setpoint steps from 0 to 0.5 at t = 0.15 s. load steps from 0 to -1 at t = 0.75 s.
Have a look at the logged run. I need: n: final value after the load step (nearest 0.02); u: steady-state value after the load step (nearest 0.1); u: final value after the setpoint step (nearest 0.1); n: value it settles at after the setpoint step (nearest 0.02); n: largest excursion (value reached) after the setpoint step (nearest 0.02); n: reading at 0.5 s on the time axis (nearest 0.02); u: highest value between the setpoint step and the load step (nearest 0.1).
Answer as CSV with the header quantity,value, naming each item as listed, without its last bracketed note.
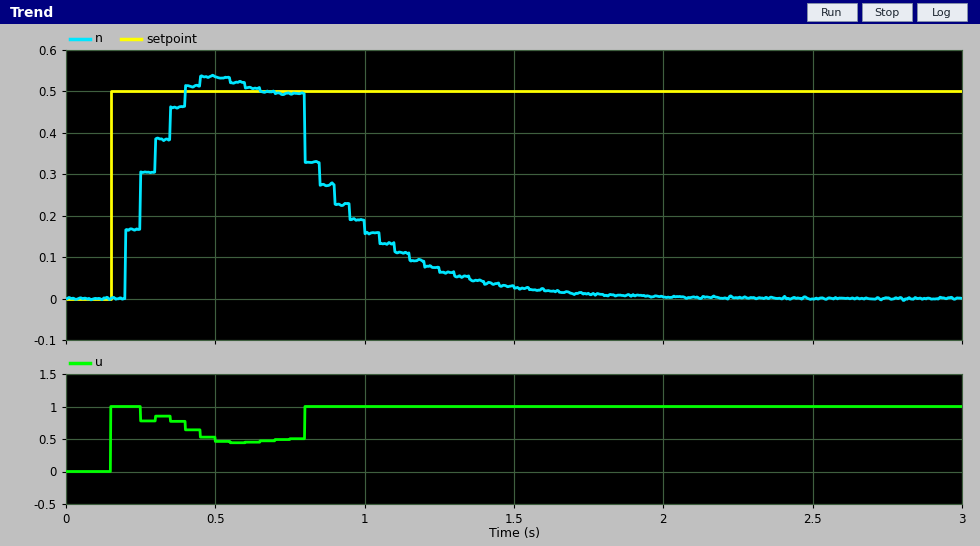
quantity,value
n: final value after the load step,0.00
u: steady-state value after the load step,1.0
u: final value after the setpoint step,0.5
n: value it settles at after the setpoint step,0.50
n: largest excursion (value reached) after the setpoint step,0.54
n: reading at 0.5 s on the time axis,0.54
u: highest value between the setpoint step and the load step,1.0
